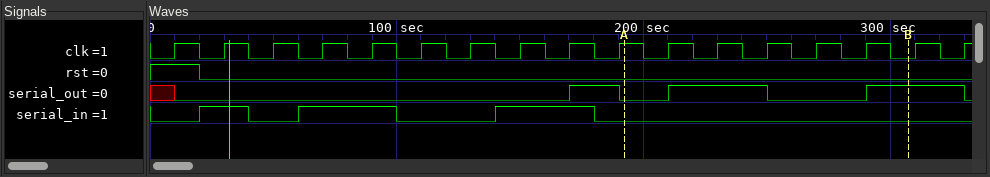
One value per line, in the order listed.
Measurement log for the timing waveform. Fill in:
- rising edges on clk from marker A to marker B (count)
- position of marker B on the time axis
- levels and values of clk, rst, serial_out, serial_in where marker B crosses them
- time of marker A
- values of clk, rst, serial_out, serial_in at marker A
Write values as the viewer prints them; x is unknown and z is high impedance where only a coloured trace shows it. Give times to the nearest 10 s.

5
310 s
clk=0, rst=0, serial_out=1, serial_in=0
190 s
clk=1, rst=0, serial_out=0, serial_in=0
